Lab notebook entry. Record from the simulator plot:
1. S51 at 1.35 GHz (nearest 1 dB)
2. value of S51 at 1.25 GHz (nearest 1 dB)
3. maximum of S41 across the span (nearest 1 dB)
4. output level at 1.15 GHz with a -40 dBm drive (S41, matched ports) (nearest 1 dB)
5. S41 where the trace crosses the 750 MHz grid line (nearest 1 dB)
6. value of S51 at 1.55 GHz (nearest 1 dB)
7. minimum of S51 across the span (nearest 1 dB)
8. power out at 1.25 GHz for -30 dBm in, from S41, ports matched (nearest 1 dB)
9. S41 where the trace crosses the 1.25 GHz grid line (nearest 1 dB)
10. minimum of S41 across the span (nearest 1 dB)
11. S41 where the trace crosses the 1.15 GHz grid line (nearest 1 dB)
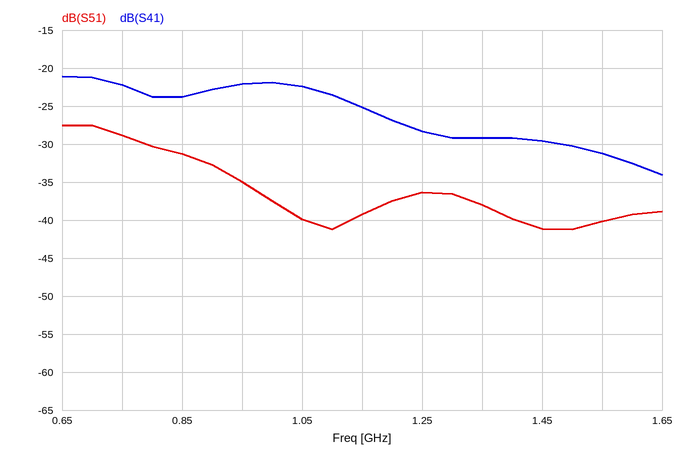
-38 dB
-36 dB
-21 dB
-65 dBm
-22 dB
-40 dB
-41 dB
-58 dBm
-28 dB
-34 dB
-25 dB
